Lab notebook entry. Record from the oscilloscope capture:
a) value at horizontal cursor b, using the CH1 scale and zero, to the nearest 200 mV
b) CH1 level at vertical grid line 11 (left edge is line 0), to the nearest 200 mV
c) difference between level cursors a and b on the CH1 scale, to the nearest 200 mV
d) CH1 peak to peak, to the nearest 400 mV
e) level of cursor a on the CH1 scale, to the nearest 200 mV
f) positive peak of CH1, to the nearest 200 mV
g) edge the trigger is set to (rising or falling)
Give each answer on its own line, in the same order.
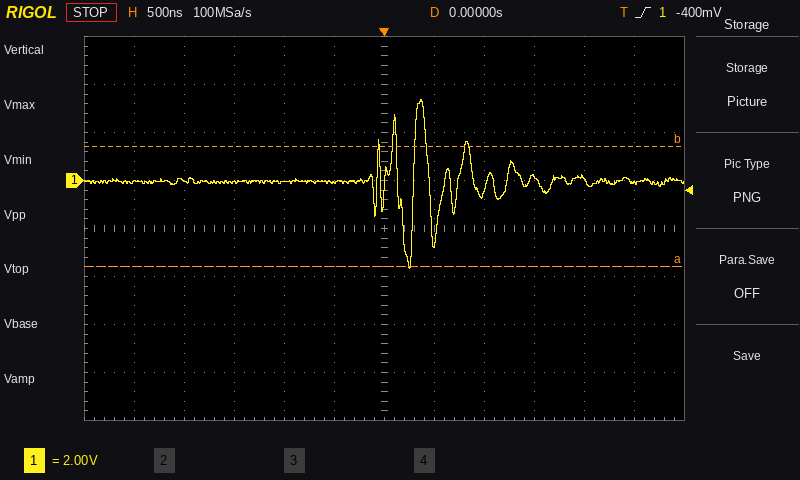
1.4 V
-200 mV
5.0 V
7.2 V
-3.6 V
3.4 V
rising
